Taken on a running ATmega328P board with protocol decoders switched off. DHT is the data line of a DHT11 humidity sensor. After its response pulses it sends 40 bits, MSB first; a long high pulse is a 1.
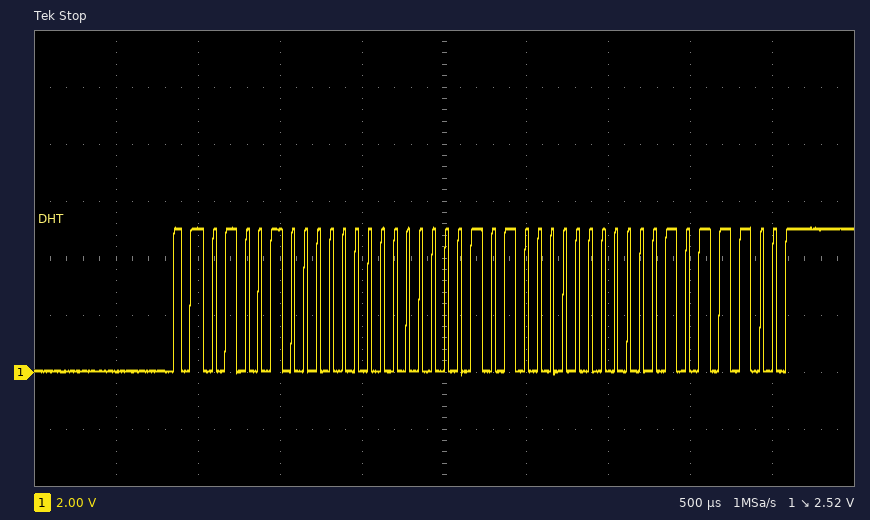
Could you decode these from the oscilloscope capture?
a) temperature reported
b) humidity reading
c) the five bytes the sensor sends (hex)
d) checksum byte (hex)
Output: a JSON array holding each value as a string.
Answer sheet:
["20.0 °C", "72 %", "48 00 14 00 5C", "0x5C"]
